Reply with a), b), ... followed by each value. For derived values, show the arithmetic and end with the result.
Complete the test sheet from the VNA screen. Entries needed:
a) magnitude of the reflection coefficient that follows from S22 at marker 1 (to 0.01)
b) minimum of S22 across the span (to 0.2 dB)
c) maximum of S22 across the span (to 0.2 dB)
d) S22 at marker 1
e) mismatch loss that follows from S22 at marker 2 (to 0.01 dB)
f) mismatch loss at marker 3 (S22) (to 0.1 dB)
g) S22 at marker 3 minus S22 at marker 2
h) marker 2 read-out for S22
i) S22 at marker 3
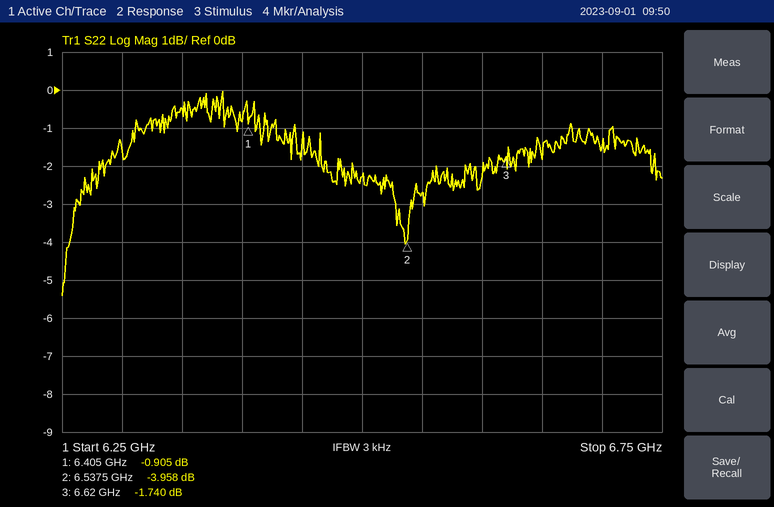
a) 10^(-0.905/20) ≈ 0.90
b) -5.4 dB
c) 0.0 dB
d) -0.905 dB
e) −10 log10(1 − 10^(-3.958/10)) ≈ 2.23 dB
f) −10 log10(1 − 10^(-1.74/10)) ≈ 4.8 dB
g) -1.74 − (-3.958) = 2.218 dB
h) -3.958 dB
i) -1.740 dB
